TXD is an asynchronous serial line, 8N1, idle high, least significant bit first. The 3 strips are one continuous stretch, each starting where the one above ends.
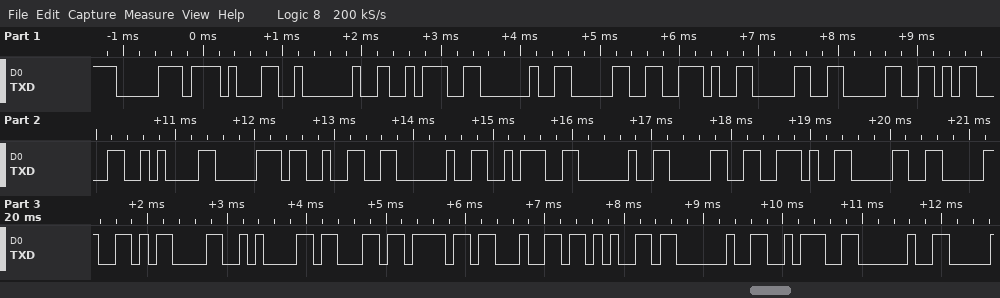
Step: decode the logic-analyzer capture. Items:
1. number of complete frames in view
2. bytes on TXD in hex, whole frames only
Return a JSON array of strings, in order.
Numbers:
["29", "70 31 20 3A 20 30 2E 30 30 0D 0A 70 32 20 3A 20 30 2E 30 30 0D 0A 63 6F 64 65 20 3A 20"]
